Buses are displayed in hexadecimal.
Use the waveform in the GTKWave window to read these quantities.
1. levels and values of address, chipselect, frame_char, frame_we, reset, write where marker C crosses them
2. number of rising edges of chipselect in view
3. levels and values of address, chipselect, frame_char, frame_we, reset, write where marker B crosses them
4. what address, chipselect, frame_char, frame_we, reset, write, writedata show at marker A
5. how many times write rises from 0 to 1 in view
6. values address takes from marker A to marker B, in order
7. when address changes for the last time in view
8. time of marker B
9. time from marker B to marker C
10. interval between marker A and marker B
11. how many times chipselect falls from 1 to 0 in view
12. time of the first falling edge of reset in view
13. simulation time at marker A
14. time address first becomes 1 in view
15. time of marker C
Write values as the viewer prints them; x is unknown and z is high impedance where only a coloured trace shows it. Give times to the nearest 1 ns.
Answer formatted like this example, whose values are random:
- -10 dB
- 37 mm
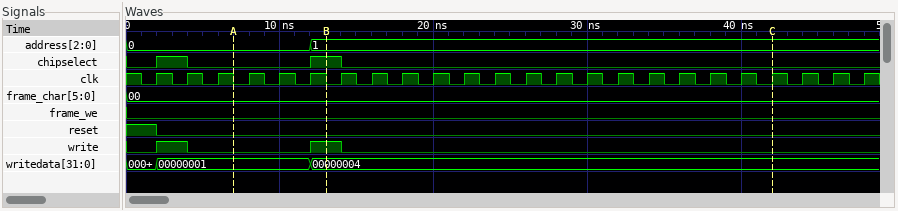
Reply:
- address=1, chipselect=0, frame_char=00, frame_we=0, reset=0, write=0
- 2
- address=1, chipselect=1, frame_char=00, frame_we=0, reset=0, write=1
- address=0, chipselect=0, frame_char=00, frame_we=0, reset=0, write=0, writedata=00000001
- 2
- 0, 1
- 12 ns
- 13 ns
- 29 ns
- 6 ns
- 2
- 2 ns
- 7 ns
- 12 ns
- 42 ns
